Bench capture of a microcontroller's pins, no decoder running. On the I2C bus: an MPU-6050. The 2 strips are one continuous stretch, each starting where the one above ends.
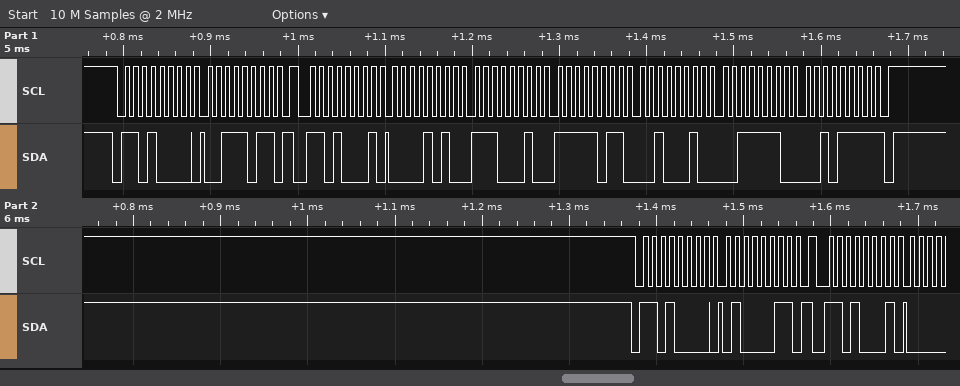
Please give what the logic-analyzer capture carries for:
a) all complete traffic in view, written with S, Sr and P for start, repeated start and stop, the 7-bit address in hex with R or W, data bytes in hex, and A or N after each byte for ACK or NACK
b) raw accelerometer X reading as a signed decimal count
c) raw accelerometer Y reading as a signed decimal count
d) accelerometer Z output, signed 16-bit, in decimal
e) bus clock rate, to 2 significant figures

S 68W A 3B A Sr 68R A 0A A E2 A FB A 22 A 3E A 2F N P S 68W A 43 A Sr 68R A
2786
-1246
15919
100 kHz
